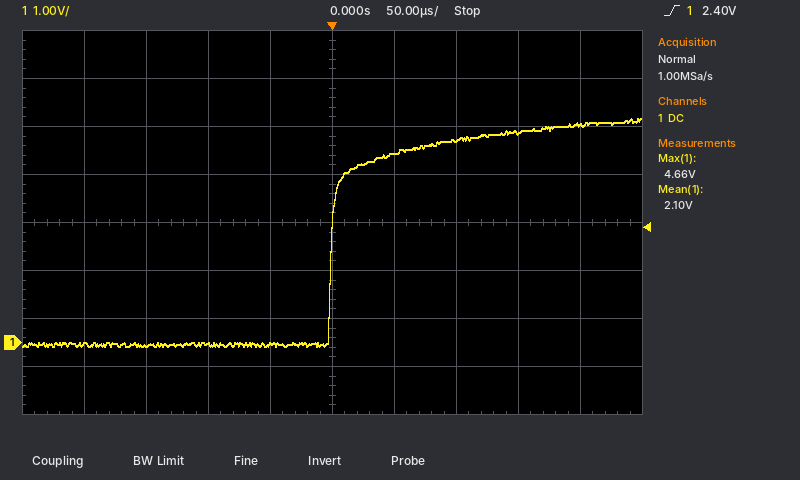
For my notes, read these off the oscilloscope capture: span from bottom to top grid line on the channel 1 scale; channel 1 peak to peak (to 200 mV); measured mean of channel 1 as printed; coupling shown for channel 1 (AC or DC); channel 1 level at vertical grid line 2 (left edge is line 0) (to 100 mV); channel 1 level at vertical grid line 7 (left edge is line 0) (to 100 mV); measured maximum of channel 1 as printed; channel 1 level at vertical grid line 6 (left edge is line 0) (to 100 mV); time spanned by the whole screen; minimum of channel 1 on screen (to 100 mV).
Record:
8 V
4.8 V
2.10 V
DC
-100 mV
4.2 V
4.66 V
3.9 V
500 µs
-100 mV
